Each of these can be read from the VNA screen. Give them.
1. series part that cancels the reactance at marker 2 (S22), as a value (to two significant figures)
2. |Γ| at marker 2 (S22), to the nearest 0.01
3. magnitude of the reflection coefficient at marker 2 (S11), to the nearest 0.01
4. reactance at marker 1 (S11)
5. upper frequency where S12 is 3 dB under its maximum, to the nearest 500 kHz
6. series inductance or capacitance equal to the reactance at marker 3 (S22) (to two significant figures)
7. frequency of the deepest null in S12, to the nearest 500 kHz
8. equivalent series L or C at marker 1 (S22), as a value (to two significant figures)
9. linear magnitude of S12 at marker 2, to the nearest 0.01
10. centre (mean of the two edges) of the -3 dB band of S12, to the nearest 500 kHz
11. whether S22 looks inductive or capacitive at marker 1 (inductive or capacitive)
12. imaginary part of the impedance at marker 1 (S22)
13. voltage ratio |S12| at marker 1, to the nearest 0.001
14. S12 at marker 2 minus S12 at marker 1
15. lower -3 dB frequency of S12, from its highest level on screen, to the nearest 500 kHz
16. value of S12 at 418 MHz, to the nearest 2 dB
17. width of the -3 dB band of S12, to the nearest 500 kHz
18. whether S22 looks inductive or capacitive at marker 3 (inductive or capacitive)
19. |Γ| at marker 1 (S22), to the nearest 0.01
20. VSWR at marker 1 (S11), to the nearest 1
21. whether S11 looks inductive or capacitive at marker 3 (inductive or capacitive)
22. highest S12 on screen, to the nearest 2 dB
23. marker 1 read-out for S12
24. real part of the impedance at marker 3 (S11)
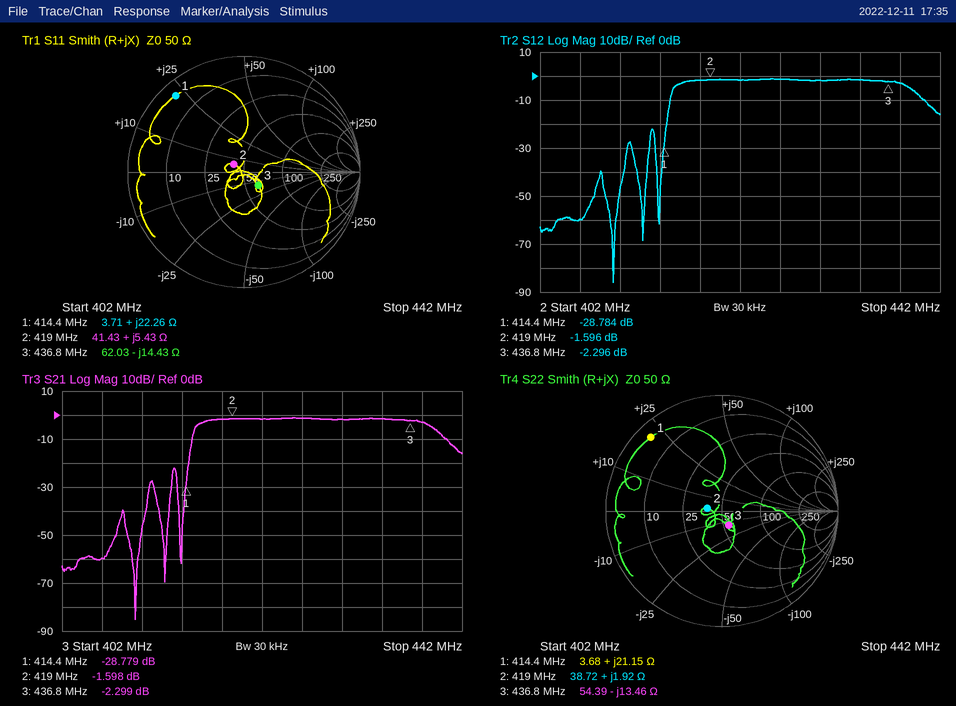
200 pF
0.13
0.11
+22.26 Ω
438.5 MHz
27 pF
409.5 MHz
8.1 nH
0.83
427.0 MHz
inductive
+21.15 Ω
0.036
27.188 dB
415.5 MHz
-2 dB
23.0 MHz
capacitive
0.88
16
capacitive
-2 dB
-28.784 dB
62.03 Ω
